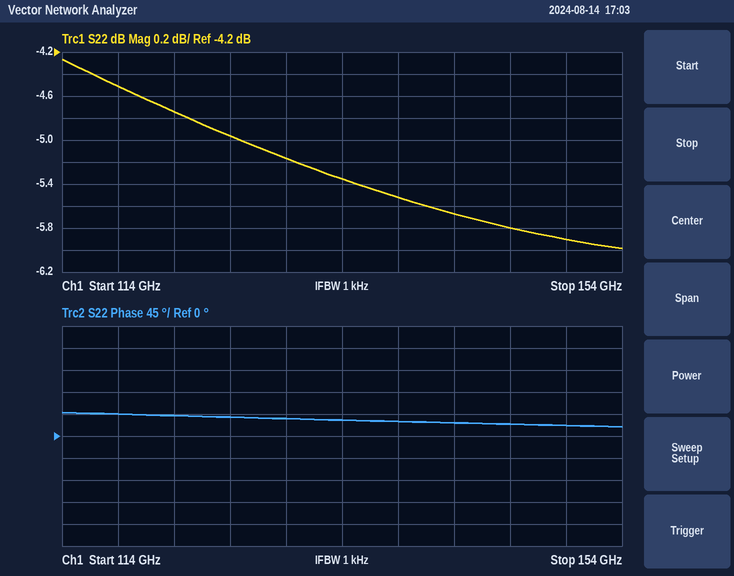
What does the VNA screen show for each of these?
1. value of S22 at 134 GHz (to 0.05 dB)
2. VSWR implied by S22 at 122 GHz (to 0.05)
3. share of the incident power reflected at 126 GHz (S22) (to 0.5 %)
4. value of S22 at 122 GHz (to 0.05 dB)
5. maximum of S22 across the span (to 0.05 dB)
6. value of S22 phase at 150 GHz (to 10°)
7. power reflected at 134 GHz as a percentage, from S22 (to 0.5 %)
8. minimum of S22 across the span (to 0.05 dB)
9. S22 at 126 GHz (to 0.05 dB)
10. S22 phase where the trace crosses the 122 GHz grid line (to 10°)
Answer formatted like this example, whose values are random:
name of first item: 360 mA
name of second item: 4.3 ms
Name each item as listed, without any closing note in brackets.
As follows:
value of S22 at 134 GHz: -5.35 dB
VSWR implied by S22 at 122 GHz: 3.75
share of the incident power reflected at 126 GHz (S22): 32.0 %
value of S22 at 122 GHz: -4.75 dB
maximum of S22 across the span: -4.25 dB
value of S22 phase at 150 GHz: 20°
power reflected at 134 GHz as a percentage, from S22: 29.0 %
minimum of S22 across the span: -6.00 dB
S22 at 126 GHz: -4.95 dB
S22 phase where the trace crosses the 122 GHz grid line: 40°
